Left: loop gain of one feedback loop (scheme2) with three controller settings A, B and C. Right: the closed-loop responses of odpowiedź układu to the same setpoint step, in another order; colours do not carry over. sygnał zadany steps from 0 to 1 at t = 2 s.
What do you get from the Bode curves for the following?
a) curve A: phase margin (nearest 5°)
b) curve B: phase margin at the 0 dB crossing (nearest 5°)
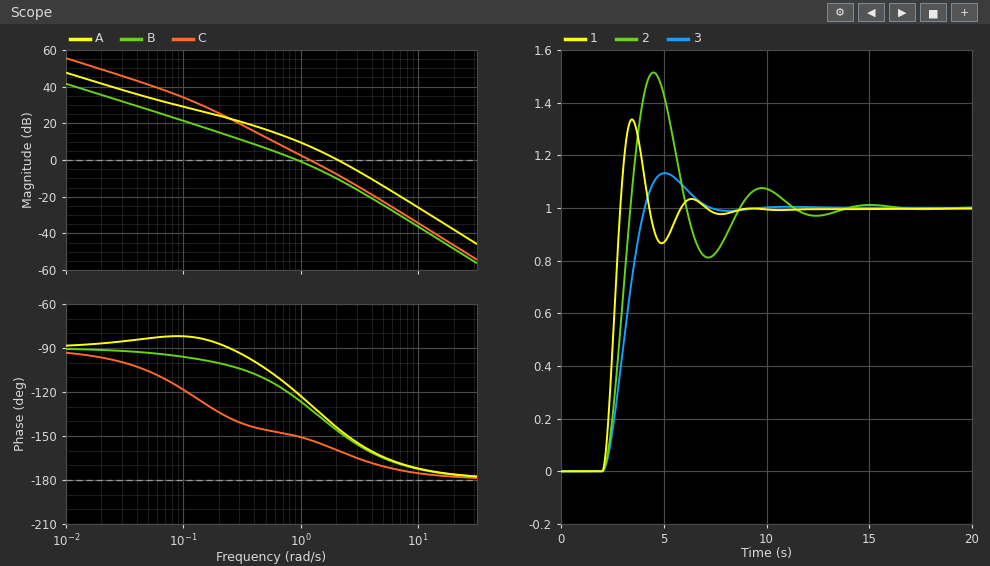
35°
55°
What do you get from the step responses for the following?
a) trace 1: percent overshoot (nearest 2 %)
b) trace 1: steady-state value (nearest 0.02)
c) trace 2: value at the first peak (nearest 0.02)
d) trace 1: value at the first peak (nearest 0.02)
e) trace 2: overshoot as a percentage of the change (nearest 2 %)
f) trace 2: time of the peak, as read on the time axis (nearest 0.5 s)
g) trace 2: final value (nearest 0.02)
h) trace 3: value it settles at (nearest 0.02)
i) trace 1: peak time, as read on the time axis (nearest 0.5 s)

34 %
1.00
1.52
1.34
52 %
4.5 s
1.00
1.00
3.5 s
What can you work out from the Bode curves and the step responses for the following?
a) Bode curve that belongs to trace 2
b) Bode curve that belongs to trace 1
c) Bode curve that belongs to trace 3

C
A
B
